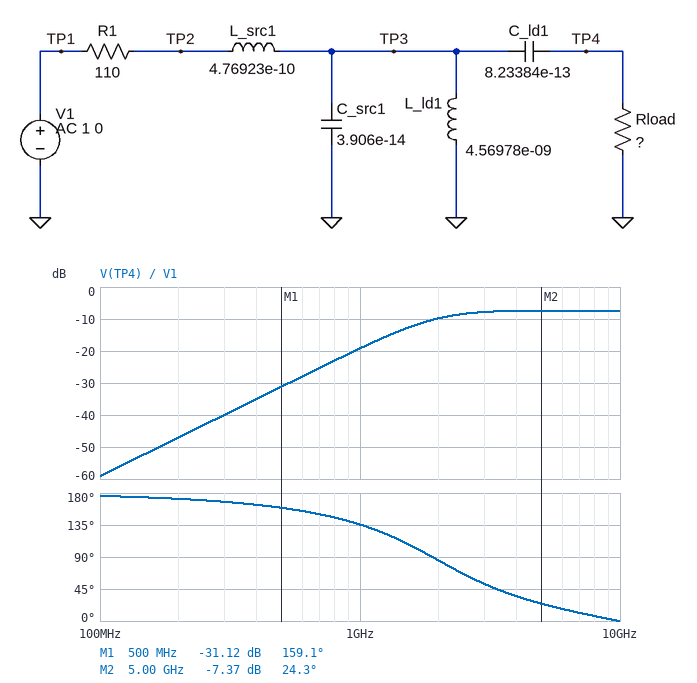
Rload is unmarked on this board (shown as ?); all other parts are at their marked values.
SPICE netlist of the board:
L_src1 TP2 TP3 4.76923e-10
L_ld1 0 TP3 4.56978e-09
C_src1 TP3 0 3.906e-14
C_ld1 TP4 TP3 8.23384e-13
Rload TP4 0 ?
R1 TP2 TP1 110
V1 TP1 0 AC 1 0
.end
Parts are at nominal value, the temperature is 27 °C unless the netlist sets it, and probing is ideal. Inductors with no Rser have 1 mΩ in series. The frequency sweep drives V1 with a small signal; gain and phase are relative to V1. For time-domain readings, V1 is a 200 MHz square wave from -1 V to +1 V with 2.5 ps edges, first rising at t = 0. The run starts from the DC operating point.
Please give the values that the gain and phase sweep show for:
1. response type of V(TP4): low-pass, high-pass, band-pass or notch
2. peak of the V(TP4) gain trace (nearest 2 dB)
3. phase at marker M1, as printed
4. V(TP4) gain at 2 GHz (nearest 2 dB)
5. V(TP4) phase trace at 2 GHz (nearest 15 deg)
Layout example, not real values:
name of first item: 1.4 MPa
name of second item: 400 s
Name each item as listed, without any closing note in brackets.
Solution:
response type of V(TP4): low-pass, high-pass, band-pass or notch: high-pass
peak of the V(TP4) gain trace: -8 dB
phase at marker M1, as printed: 159.1 deg
V(TP4) gain at 2 GHz: -10 dB
V(TP4) phase trace at 2 GHz: 90 deg
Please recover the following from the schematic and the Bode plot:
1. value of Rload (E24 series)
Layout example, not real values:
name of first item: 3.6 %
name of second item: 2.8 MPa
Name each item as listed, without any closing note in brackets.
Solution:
value of Rload: 82 Ω
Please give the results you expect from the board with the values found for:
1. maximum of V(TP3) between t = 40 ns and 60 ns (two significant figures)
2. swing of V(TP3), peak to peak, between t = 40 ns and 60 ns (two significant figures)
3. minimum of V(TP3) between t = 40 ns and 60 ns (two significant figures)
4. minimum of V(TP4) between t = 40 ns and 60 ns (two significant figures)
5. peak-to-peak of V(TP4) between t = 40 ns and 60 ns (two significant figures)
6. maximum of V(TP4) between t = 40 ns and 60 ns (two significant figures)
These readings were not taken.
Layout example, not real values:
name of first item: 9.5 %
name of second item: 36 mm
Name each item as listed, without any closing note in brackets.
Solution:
maximum of V(TP3) between t = 40 ns and 60 ns: 860 mV
swing of V(TP3), peak to peak, between t = 40 ns and 60 ns: 1.7 V
minimum of V(TP3) between t = 40 ns and 60 ns: -860 mV
minimum of V(TP4) between t = 40 ns and 60 ns: -770 mV
peak-to-peak of V(TP4) between t = 40 ns and 60 ns: 1.5 V
maximum of V(TP4) between t = 40 ns and 60 ns: 770 mV
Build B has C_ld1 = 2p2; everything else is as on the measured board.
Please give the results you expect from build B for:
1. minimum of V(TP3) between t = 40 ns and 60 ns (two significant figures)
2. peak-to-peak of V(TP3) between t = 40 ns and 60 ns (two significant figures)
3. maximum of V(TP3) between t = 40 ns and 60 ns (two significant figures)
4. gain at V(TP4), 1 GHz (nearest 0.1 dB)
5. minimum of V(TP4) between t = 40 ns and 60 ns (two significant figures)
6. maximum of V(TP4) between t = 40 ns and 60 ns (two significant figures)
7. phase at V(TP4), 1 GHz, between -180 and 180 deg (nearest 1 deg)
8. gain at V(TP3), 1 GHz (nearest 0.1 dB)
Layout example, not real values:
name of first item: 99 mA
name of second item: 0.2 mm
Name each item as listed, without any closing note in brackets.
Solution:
minimum of V(TP3) between t = 40 ns and 60 ns: -830 mV
peak-to-peak of V(TP3) between t = 40 ns and 60 ns: 1.7 V
maximum of V(TP3) between t = 40 ns and 60 ns: 830 mV
gain at V(TP4), 1 GHz: -13.7 dB
minimum of V(TP4) between t = 40 ns and 60 ns: -800 mV
maximum of V(TP4) between t = 40 ns and 60 ns: 800 mV
phase at V(TP4), 1 GHz, between -180 and 180 deg: 101 deg
gain at V(TP3), 1 GHz: -11.2 dB
